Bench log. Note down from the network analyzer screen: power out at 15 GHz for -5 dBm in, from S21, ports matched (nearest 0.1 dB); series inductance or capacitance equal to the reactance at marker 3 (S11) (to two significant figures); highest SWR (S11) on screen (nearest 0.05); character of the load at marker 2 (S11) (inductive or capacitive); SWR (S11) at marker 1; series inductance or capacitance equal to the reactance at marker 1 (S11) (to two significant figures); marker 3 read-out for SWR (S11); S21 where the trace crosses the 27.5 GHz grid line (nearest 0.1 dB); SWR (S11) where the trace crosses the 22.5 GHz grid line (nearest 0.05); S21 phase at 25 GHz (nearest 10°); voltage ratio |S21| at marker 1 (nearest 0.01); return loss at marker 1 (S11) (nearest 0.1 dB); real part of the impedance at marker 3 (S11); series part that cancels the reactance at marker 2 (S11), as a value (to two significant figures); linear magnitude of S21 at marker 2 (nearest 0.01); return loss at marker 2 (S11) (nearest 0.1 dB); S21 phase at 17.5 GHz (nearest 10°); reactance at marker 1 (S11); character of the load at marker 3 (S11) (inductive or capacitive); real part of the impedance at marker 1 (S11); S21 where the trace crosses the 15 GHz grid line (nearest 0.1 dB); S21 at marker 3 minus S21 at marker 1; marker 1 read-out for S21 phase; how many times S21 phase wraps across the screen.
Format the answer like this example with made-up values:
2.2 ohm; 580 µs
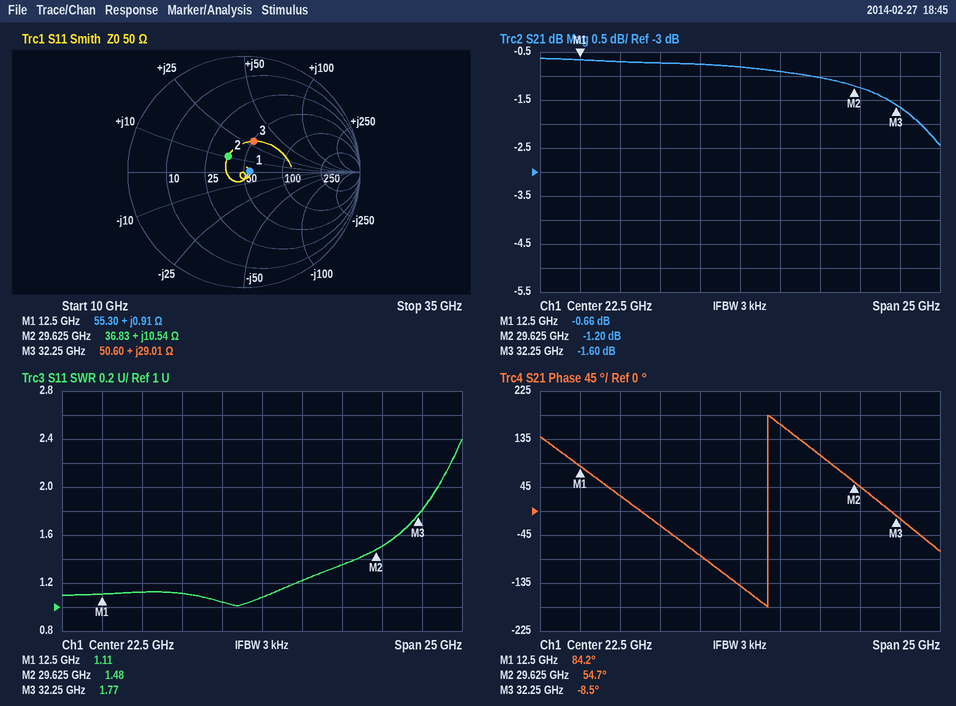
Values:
-5.7 dBm; 140 pH; 2.40; inductive; 1.11; 12 pH; 1.77; -1.0 dB; 1.10; 160°; 0.93; 25.8 dB; 50.60 Ω; 510 fF; 0.87; 14.3 dB; -30°; +0.91 Ω; inductive; 55.30 Ω; -0.7 dB; -0.94 dB; 84.2°; 1
